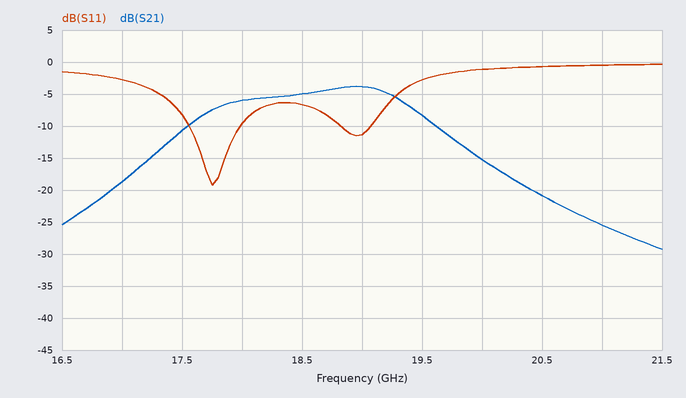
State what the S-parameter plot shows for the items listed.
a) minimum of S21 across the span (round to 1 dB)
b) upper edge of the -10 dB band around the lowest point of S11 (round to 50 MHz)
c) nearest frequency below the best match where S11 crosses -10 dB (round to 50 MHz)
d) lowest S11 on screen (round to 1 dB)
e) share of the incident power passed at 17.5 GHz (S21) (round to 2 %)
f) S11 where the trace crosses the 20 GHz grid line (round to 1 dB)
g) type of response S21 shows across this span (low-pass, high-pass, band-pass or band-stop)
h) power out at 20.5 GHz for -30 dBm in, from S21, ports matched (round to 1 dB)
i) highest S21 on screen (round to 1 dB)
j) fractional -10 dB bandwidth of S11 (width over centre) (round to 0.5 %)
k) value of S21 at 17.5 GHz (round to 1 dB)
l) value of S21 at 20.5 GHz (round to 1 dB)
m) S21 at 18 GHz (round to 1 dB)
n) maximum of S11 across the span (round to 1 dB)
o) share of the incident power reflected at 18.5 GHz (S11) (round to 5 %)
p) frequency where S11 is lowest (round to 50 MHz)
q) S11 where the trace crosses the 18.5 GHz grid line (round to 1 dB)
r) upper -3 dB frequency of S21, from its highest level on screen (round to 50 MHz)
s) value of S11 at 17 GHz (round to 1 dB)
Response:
-29 dB
18.00 GHz
17.55 GHz
-19 dB
8 %
-1 dB
band-pass
-51 dBm
-4 dB
2.5 %
-11 dB
-21 dB
-6 dB
0 dB
20 %
17.75 GHz
-7 dB
19.40 GHz
-3 dB
